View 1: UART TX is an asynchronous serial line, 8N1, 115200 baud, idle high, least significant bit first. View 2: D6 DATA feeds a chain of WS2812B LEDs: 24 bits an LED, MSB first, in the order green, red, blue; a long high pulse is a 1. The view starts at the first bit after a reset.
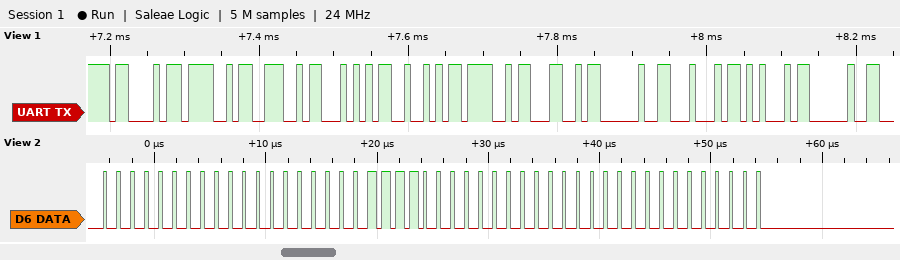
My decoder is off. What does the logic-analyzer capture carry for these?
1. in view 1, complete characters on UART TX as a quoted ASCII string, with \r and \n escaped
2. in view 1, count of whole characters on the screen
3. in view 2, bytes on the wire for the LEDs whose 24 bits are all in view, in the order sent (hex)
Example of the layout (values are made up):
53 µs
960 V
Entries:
"CONTROL DE "
11
00 00 1E 00 00 00
